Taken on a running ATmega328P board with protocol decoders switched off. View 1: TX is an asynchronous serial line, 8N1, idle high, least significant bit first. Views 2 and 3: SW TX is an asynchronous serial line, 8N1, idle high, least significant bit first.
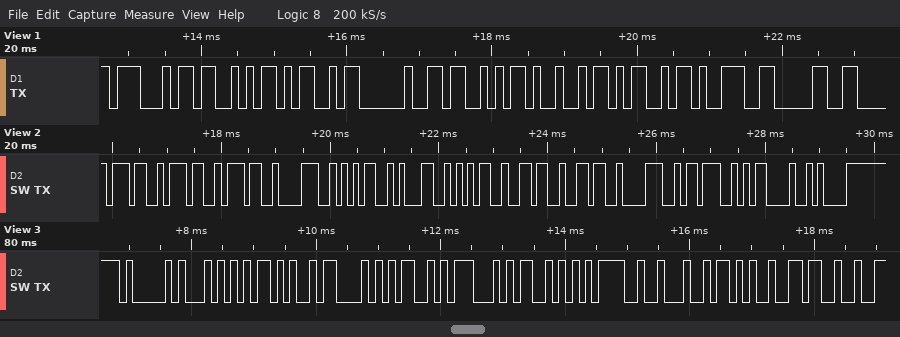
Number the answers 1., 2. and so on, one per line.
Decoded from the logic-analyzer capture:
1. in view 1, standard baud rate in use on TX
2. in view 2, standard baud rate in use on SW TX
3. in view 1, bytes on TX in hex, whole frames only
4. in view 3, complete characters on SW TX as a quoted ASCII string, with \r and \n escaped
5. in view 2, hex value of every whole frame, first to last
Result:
1. 9600 baud
2. 9600 baud
3. 47 53 4D 20 53 49 4D 39 30
4. "AT+CMGS=\"+6"
5. 37 37 37 38 35 31 35 36 36 38 3B 0D 0A
